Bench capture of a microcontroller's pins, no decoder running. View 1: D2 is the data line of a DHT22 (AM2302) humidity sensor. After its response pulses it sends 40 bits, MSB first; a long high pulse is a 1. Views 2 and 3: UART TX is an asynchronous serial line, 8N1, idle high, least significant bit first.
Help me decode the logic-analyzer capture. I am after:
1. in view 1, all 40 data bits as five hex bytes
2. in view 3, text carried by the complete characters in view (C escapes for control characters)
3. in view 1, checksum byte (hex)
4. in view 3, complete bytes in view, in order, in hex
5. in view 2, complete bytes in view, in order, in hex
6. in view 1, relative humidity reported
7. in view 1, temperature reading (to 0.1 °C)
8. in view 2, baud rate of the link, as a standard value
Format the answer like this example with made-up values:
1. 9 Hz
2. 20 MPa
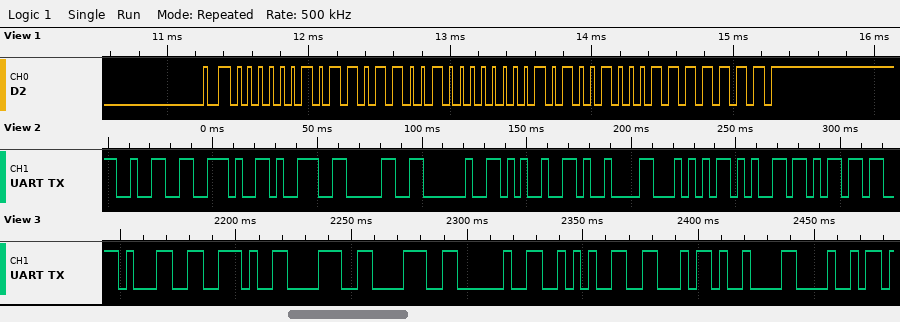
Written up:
1. 02 D9 00 A4 7F
2. "1.88 *F\tH"
3. 0x7F
4. 31 2E 38 38 20 2A 46 09 48
5. 32 2E 39 30 20 25 09 54 65 6D
6. 72.9 %
7. 16.4 °C
8. 300 baud
